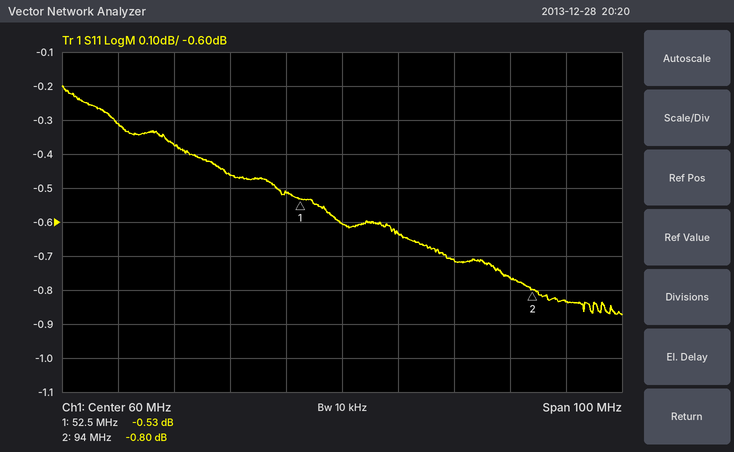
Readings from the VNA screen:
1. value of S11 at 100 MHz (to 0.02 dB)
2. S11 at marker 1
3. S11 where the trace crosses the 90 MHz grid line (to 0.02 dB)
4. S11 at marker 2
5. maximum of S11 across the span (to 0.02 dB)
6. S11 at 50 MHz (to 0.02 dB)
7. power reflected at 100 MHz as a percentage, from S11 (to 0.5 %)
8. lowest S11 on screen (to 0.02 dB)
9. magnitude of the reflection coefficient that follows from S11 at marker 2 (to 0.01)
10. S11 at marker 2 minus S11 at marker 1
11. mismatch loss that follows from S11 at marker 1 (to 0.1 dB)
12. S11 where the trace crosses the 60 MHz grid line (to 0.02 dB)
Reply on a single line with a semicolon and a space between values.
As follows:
-0.84 dB; -0.53 dB; -0.76 dB; -0.80 dB; -0.20 dB; -0.52 dB; 82.5 %; -0.88 dB; 0.91; -0.27 dB; 9.4 dB; -0.60 dB
